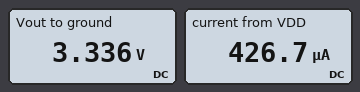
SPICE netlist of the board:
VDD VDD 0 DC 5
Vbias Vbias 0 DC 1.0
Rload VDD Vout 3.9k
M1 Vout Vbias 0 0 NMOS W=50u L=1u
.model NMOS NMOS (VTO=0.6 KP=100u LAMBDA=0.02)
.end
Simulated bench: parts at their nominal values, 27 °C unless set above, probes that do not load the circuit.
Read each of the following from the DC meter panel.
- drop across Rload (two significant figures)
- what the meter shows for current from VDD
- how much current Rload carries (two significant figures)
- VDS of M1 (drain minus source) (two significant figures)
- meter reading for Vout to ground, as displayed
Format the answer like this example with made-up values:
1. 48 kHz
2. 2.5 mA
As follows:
1. 1.7 V
2. 426.7 µA
3. 430 µA
4. 3.3 V
5. 3.336 V
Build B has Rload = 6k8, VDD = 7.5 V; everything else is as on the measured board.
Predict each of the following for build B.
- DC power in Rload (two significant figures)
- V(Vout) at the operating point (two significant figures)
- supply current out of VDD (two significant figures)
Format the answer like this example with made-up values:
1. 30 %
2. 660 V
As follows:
1. 1.3 mW
2. 4.5 V
3. 440 µA
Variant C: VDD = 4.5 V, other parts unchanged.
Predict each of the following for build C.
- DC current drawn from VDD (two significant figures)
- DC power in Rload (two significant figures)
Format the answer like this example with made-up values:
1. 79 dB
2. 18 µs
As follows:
1. 420 µA
2. 700 µW
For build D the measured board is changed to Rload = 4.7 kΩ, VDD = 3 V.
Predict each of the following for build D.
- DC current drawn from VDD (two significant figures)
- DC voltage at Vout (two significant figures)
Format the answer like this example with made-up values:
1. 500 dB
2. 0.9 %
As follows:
1. 410 µA
2. 1.1 V
